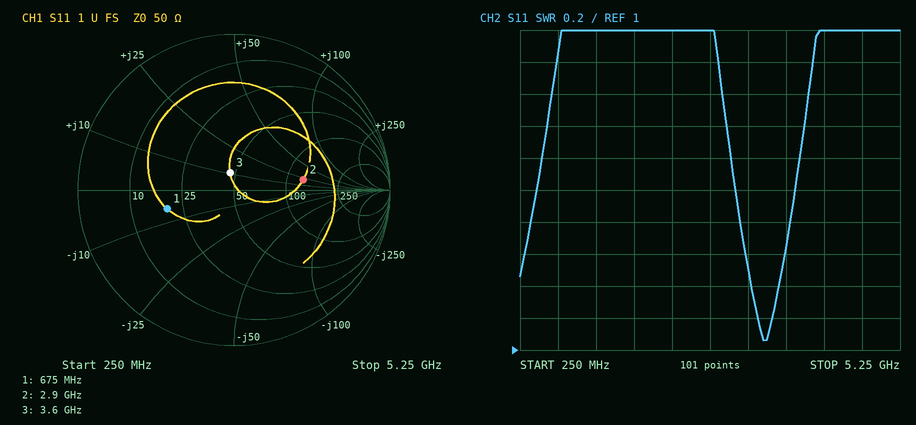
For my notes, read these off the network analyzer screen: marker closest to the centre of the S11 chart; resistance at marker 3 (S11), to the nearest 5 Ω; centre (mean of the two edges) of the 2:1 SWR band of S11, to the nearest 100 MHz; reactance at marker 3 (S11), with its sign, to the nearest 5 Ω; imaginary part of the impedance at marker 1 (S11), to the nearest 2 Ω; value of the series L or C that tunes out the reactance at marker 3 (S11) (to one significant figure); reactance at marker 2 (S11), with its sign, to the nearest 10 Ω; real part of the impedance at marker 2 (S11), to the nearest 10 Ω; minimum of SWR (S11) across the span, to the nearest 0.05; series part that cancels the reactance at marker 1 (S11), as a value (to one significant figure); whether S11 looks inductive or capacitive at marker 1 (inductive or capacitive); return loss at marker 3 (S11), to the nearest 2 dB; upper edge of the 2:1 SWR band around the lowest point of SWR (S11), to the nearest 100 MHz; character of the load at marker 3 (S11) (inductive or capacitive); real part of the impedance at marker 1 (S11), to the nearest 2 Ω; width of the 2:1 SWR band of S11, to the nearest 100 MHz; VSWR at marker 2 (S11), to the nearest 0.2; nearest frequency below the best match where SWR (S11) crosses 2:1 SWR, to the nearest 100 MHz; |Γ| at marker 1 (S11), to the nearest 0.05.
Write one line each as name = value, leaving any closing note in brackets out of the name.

marker closest to the centre of the S11 chart = marker 3
resistance at marker 3 (S11), to the nearest 5 Ω = 45 Ω
centre (mean of the two edges) of the 2:1 SWR band of S11, to the nearest 100 MHz = 3.5 GHz
reactance at marker 3 (S11), with its sign, to the nearest 5 Ω = +10 Ω
imaginary part of the impedance at marker 1 (S11), to the nearest 2 Ω = -6 Ω
value of the series L or C that tunes out the reactance at marker 3 (S11) = 4 pF
reactance at marker 2 (S11), with its sign, to the nearest 10 Ω = +20 Ω
real part of the impedance at marker 2 (S11), to the nearest 10 Ω = 130 Ω
minimum of SWR (S11) across the span, to the nearest 0.05 = 1.05
series part that cancels the reactance at marker 1 (S11), as a value = 1 nH
whether S11 looks inductive or capacitive at marker 1 = capacitive
return loss at marker 3 (S11), to the nearest 2 dB = 18 dB
upper edge of the 2:1 SWR band around the lowest point of SWR (S11), to the nearest 100 MHz = 3.9 GHz
character of the load at marker 3 (S11) = inductive
real part of the impedance at marker 1 (S11), to the nearest 2 Ω = 20 Ω
width of the 2:1 SWR band of S11, to the nearest 100 MHz = 800 MHz
VSWR at marker 2 (S11), to the nearest 0.2 = 2.6
nearest frequency below the best match where SWR (S11) crosses 2:1 SWR, to the nearest 100 MHz = 3.1 GHz
|Γ| at marker 1 (S11), to the nearest 0.05 = 0.45
